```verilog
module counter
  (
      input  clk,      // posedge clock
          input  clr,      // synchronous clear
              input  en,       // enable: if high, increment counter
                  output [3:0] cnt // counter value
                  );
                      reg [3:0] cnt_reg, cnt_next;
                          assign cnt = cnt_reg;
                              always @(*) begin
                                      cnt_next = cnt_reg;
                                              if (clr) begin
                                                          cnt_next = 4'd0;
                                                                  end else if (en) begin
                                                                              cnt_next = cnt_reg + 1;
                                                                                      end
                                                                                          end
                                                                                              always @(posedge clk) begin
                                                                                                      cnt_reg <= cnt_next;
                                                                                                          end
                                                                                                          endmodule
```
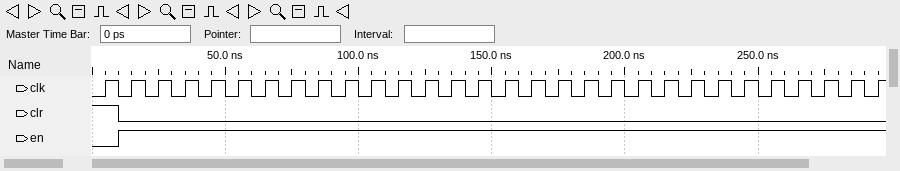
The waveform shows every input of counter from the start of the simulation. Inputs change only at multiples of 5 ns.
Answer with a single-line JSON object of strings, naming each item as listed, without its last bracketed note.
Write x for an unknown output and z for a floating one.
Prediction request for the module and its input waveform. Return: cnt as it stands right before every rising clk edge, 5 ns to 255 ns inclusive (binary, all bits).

{"cnt as it stands right before every rising clk edge, 5 ns to 255 ns inclusive": "x, 0000, 0001, 0010, 0011, 0100, 0101, 0110, 0111, 1000, 1001, 1010, 1011, 1100, 1101, 1110, 1111, 0000, 0001, 0010, 0011, 0100, 0101, 0110, 0111, 1000"}
